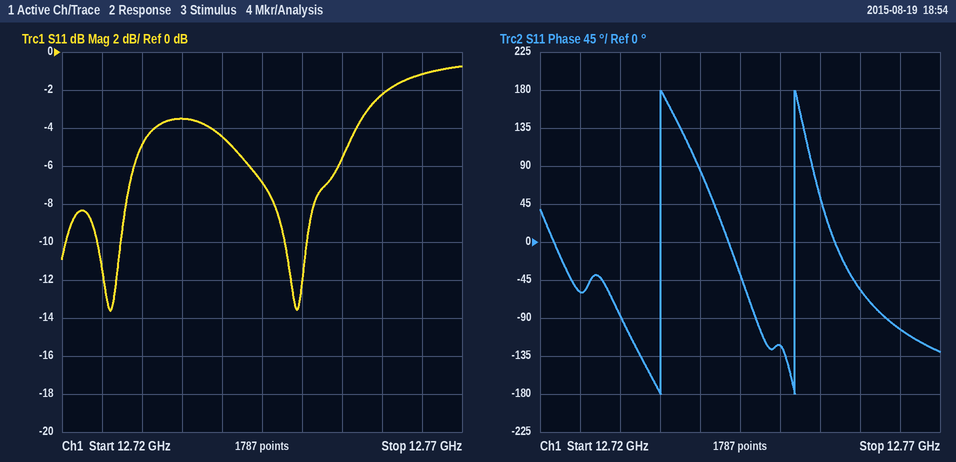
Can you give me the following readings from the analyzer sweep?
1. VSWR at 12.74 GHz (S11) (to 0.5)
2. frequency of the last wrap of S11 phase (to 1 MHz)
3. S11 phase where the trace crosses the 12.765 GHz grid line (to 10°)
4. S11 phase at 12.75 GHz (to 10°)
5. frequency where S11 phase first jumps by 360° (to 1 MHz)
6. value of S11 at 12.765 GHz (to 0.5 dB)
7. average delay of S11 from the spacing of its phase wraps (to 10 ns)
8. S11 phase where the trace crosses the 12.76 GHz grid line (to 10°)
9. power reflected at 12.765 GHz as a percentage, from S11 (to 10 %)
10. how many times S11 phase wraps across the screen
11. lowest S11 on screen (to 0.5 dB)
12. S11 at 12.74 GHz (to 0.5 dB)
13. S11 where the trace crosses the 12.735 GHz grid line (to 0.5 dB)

4.0
12.752 GHz
-100°
-120°
12.735 GHz
-1.0 dB
60 ns
-60°
80 %
2
-13.5 dB
-4.5 dB
-3.5 dB
